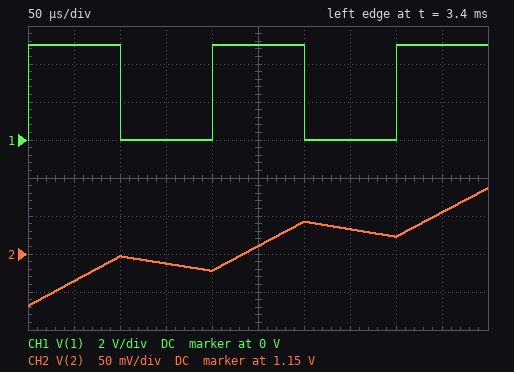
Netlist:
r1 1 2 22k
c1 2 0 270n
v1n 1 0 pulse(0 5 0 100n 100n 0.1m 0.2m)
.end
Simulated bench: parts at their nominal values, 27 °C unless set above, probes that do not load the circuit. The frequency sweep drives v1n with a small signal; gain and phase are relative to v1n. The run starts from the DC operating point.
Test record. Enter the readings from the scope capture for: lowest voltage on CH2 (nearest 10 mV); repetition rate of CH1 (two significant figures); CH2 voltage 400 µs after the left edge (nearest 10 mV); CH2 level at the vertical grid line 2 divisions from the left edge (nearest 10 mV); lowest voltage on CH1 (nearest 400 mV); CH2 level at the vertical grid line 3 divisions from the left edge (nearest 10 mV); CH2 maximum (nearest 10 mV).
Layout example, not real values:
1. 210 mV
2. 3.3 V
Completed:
1. 1.08 V
2. 5.0 kHz
3. 1.17 V
4. 1.15 V
5. 0 V
6. 1.14 V
7. 1.24 V
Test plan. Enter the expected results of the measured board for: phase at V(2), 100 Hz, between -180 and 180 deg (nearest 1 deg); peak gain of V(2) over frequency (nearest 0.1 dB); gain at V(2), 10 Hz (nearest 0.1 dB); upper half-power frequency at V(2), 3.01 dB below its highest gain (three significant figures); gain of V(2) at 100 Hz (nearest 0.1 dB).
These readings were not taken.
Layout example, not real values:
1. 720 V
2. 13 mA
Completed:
1. -75 deg
2. 0 dB
3. -0.6 dB
4. 26.8 Hz
5. -11.7 dB
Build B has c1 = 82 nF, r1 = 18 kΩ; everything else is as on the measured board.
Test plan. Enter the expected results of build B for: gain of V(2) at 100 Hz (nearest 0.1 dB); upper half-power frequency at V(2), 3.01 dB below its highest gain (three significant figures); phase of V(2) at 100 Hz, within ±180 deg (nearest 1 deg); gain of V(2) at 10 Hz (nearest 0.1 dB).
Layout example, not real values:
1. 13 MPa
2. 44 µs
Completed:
1. -2.7 dB
2. 108 Hz
3. -43 deg
4. 0 dB
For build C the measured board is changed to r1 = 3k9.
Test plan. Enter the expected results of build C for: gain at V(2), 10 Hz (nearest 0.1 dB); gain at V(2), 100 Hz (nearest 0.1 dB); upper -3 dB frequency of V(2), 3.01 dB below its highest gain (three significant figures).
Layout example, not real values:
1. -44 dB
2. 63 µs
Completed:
1. 0 dB
2. -1.6 dB
3. 151 Hz
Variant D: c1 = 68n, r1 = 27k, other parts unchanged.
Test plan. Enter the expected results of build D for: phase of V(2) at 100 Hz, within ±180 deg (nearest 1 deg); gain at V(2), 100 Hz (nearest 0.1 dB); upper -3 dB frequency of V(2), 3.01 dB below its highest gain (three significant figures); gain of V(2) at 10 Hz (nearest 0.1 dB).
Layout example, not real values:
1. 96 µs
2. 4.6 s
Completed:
1. -49 deg
2. -3.7 dB
3. 86.7 Hz
4. -0.1 dB
